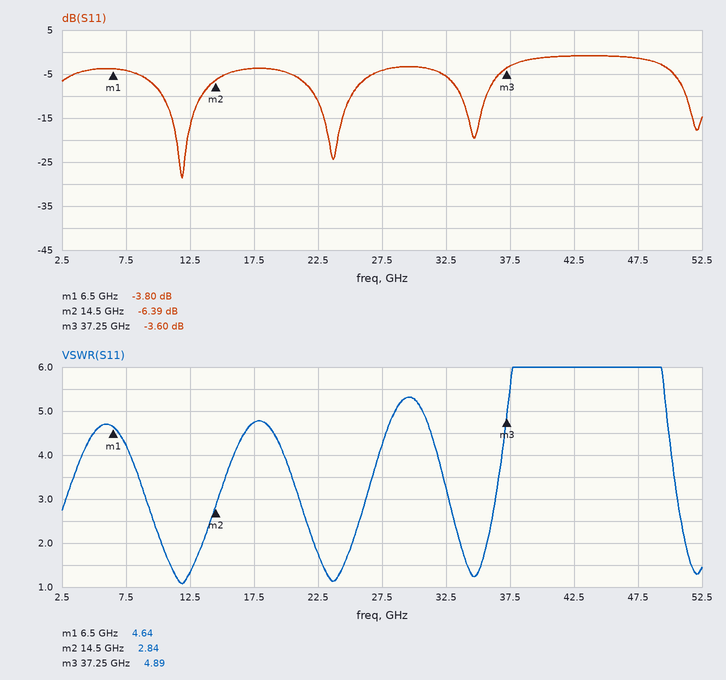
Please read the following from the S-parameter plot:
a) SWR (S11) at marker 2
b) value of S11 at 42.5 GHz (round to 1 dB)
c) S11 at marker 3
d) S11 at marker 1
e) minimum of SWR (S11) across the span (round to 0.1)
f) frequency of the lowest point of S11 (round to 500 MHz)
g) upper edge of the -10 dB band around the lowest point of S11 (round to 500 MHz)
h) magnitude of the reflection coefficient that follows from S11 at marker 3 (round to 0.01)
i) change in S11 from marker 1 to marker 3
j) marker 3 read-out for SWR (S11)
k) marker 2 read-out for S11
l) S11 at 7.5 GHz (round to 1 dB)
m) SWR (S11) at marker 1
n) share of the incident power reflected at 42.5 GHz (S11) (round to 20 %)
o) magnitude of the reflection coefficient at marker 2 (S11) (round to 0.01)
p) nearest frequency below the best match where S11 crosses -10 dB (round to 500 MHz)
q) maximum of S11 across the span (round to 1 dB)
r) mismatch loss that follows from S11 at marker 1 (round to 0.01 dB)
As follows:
2.84
-1 dB
-3.60 dB
-3.80 dB
1.1
12.0 GHz
13.5 GHz
0.66
0.20 dB
4.89
-6.39 dB
-4 dB
4.64
80 %
0.48
10.5 GHz
-1 dB
2.34 dB
